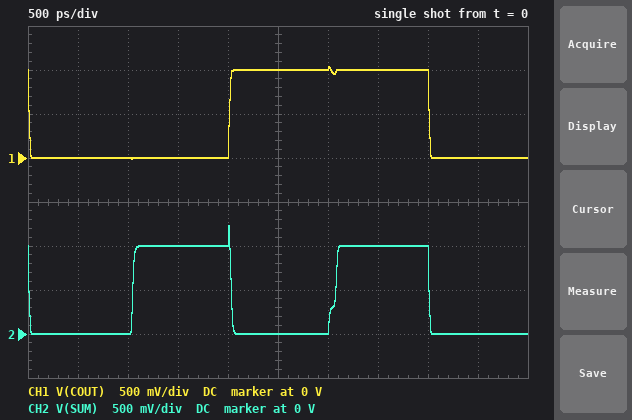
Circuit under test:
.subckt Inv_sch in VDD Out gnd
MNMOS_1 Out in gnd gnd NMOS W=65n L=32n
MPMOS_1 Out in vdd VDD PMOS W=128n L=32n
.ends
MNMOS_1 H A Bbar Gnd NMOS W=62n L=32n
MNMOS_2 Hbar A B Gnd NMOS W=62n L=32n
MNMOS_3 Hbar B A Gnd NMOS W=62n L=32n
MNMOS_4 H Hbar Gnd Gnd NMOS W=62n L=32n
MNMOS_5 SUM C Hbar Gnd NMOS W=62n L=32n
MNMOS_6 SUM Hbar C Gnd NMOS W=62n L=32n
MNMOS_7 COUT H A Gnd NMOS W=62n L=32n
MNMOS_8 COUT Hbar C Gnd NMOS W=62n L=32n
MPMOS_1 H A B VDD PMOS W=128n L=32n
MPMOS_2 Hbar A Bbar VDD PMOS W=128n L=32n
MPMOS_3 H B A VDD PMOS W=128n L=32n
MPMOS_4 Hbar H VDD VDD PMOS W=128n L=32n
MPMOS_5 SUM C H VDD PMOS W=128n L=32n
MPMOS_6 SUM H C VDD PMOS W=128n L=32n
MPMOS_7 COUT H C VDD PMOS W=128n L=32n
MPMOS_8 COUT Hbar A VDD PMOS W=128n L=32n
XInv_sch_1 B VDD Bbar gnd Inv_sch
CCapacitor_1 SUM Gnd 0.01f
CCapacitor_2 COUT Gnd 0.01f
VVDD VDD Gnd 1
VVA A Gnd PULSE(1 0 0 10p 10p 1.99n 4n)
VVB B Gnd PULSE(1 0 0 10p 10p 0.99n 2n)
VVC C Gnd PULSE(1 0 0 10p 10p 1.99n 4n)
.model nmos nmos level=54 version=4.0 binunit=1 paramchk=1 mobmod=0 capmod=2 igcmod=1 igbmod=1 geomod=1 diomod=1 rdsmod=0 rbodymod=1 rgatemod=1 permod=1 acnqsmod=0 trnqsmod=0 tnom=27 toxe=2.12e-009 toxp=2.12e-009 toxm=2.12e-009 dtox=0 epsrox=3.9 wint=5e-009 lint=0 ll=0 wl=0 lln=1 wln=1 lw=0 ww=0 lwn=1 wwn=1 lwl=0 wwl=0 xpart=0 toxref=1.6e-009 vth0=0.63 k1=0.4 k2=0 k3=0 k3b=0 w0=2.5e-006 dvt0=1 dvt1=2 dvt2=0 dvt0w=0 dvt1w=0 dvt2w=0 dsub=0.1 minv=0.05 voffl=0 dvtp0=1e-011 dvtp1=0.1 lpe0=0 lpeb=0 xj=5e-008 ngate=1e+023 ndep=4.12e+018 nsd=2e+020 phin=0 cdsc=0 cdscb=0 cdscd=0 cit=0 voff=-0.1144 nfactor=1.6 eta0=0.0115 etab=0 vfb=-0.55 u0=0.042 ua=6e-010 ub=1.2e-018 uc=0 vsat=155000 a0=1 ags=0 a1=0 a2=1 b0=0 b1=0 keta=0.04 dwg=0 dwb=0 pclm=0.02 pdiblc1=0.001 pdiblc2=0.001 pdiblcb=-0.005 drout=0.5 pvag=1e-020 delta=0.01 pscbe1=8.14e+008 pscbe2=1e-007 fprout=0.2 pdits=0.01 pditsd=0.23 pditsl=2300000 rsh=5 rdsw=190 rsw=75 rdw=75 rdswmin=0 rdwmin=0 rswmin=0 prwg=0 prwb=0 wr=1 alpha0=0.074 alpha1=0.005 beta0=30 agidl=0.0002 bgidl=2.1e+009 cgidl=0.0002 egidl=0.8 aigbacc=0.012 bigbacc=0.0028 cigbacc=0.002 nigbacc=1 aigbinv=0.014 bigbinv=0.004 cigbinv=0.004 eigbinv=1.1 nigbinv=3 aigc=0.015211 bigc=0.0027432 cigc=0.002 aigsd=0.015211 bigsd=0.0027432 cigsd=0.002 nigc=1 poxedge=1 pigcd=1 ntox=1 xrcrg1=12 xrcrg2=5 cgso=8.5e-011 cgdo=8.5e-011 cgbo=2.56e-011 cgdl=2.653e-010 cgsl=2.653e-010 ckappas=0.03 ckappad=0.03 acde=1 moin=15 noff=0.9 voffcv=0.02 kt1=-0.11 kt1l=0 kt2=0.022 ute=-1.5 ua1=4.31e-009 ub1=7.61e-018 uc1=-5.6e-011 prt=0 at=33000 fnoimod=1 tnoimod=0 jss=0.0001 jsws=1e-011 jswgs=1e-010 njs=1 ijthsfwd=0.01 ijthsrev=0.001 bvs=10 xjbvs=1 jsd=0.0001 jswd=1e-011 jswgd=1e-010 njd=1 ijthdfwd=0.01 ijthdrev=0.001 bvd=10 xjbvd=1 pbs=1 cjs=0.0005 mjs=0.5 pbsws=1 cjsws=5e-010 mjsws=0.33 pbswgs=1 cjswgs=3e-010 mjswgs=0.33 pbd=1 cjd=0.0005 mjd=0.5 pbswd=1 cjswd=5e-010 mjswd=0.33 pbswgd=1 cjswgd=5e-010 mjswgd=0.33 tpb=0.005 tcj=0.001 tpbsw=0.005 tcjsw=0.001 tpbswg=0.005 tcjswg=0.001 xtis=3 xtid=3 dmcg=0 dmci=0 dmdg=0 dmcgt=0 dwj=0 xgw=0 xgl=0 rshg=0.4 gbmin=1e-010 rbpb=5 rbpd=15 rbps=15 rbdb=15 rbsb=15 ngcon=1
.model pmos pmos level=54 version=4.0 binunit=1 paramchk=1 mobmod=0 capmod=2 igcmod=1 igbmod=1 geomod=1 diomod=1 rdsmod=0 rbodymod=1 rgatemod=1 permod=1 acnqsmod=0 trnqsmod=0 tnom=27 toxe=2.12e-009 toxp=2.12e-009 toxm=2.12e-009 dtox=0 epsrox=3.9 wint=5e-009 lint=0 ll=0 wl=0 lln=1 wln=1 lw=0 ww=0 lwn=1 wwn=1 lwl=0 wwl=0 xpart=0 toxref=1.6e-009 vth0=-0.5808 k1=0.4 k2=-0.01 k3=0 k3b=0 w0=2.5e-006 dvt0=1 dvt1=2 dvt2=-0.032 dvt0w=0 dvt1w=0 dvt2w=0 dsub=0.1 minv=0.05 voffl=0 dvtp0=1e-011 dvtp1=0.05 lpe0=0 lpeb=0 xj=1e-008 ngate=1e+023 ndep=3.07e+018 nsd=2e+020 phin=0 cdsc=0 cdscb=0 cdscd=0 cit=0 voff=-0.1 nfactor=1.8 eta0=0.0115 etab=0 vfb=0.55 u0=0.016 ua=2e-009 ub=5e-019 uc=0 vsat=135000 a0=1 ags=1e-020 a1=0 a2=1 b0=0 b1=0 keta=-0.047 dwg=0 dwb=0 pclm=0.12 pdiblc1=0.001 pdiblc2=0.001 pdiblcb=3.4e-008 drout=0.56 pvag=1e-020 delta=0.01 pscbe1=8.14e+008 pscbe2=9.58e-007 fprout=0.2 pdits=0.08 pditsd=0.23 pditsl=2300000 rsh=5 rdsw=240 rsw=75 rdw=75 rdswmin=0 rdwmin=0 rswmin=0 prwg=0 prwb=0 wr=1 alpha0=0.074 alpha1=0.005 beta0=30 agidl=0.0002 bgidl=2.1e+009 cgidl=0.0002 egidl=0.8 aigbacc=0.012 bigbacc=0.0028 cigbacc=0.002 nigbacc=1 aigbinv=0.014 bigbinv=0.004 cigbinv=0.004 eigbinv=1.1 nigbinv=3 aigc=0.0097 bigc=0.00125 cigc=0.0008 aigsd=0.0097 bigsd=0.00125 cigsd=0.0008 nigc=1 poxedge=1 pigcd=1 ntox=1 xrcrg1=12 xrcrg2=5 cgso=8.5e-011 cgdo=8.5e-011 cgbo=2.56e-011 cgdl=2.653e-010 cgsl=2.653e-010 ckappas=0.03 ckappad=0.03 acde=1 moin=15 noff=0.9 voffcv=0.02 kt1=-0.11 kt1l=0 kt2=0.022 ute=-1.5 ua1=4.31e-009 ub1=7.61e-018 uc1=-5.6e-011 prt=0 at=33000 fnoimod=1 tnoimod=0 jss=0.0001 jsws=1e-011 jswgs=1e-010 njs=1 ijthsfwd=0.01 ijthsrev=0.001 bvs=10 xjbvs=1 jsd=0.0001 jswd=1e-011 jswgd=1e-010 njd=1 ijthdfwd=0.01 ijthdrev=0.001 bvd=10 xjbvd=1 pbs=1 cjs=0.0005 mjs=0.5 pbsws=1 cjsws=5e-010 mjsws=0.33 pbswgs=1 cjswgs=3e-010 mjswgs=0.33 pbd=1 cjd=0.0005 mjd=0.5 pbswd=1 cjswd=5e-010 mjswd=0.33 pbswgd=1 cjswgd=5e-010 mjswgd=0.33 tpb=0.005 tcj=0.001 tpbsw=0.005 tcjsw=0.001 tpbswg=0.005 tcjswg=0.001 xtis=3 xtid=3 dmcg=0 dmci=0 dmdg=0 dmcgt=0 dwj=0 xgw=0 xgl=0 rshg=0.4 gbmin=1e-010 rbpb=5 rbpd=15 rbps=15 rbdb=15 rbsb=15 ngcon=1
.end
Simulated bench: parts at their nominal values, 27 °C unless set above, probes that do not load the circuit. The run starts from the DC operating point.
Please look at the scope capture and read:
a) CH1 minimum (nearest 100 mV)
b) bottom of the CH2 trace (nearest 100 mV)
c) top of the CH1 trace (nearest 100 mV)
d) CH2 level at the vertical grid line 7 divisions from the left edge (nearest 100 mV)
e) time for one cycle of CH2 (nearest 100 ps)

0 V
0 V
1.0 V
1.0 V
2.0 ns
